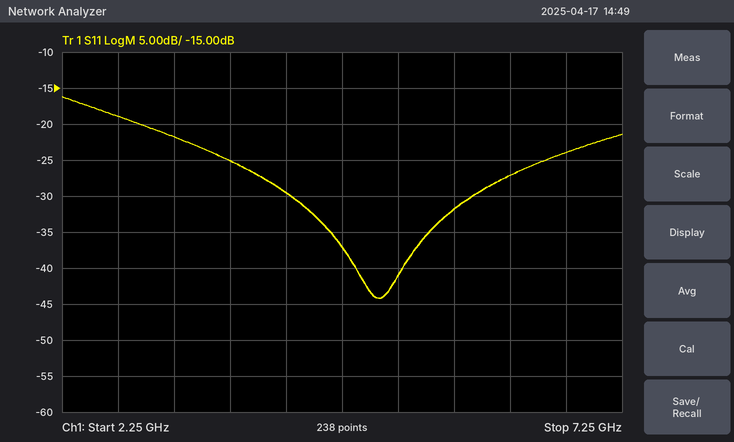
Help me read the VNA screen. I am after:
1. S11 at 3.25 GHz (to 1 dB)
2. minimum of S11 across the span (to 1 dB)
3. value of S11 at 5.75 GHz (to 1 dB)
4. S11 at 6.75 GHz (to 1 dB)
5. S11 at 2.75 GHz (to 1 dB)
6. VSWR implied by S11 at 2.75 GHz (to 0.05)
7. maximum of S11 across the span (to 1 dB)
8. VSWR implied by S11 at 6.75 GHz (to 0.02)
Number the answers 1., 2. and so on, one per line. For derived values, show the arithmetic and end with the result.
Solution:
1. -22 dB
2. -44 dB
3. -32 dB
4. -24 dB
5. -19 dB
6. |Γ| = 10^(-19/20) = 0.1122; VSWR = (1 + 0.1122)/(1 − 0.1122) ≈ 1.25
7. -16 dB
8. |Γ| = 10^(-24/20) = 0.0631; VSWR = (1 + 0.0631)/(1 − 0.0631) ≈ 1.13, so 1.14 to the nearest 0.02
